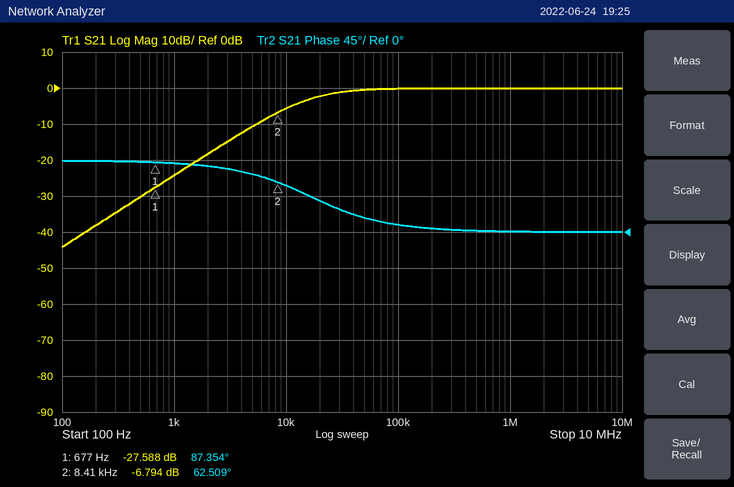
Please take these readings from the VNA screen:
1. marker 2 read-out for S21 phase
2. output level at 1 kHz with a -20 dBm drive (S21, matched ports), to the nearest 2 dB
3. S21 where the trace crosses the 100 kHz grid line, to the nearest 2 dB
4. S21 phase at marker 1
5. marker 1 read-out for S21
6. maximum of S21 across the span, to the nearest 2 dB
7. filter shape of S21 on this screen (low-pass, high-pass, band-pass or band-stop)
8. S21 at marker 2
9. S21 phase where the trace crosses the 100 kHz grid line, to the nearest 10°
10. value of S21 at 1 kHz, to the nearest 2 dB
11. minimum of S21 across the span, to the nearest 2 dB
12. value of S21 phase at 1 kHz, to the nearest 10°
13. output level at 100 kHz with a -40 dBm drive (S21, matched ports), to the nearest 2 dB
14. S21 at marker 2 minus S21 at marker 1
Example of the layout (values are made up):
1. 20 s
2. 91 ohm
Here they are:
1. 62.509°
2. -44 dBm
3. 0 dB
4. 87.354°
5. -27.588 dB
6. 0 dB
7. high-pass
8. -6.794 dB
9. 10°
10. -24 dB
11. -44 dB
12. 90°
13. -40 dBm
14. 20.794 dB
